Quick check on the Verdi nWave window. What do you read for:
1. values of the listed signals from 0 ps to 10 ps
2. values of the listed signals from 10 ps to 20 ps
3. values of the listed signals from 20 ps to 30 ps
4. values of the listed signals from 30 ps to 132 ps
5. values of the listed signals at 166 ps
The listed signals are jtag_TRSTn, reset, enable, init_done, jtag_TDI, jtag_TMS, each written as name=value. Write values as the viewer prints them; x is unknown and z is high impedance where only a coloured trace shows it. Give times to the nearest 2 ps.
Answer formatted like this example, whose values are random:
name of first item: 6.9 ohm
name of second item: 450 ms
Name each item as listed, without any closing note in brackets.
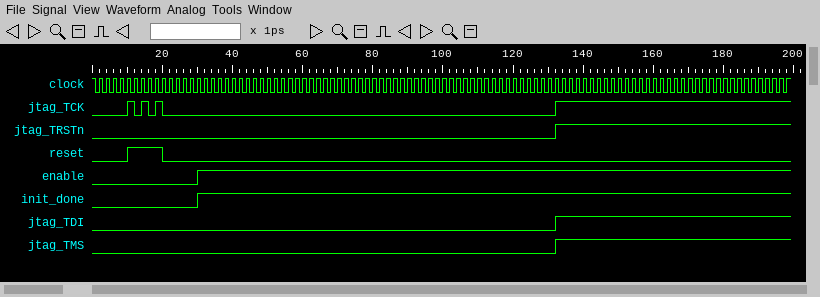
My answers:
values of the listed signals from 0 ps to 10 ps: jtag_TRSTn=0, reset=0, enable=0, init_done=0, jtag_TDI=0, jtag_TMS=0
values of the listed signals from 10 ps to 20 ps: jtag_TRSTn=0, reset=1, enable=0, init_done=0, jtag_TDI=0, jtag_TMS=0
values of the listed signals from 20 ps to 30 ps: jtag_TRSTn=0, reset=0, enable=0, init_done=0, jtag_TDI=0, jtag_TMS=0
values of the listed signals from 30 ps to 132 ps: jtag_TRSTn=0, reset=0, enable=1, init_done=1, jtag_TDI=0, jtag_TMS=0
values of the listed signals at 166 ps: jtag_TRSTn=1, reset=0, enable=1, init_done=1, jtag_TDI=1, jtag_TMS=1
